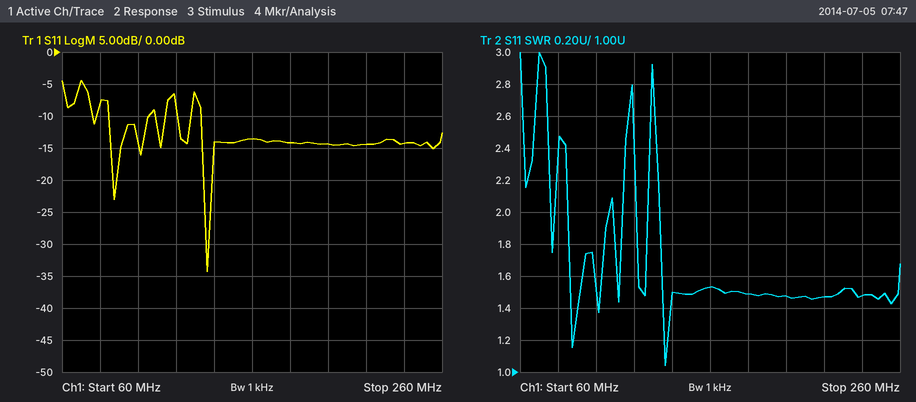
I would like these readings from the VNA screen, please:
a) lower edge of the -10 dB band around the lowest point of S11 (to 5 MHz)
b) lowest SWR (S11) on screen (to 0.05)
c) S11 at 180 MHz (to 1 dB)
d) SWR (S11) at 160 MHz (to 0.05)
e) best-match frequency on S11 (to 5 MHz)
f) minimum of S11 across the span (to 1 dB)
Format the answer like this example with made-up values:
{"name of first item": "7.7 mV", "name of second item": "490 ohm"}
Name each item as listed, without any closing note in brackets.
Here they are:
{"lower edge of the -10 dB band around the lowest point of S11": "135 MHz", "lowest SWR (S11) on screen": "1.05", "S11 at 180 MHz": "-14 dB", "SWR (S11) at 160 MHz": "1.55", "best-match frequency on S11": "135 MHz", "minimum of S11 across the span": "-34 dB"}
